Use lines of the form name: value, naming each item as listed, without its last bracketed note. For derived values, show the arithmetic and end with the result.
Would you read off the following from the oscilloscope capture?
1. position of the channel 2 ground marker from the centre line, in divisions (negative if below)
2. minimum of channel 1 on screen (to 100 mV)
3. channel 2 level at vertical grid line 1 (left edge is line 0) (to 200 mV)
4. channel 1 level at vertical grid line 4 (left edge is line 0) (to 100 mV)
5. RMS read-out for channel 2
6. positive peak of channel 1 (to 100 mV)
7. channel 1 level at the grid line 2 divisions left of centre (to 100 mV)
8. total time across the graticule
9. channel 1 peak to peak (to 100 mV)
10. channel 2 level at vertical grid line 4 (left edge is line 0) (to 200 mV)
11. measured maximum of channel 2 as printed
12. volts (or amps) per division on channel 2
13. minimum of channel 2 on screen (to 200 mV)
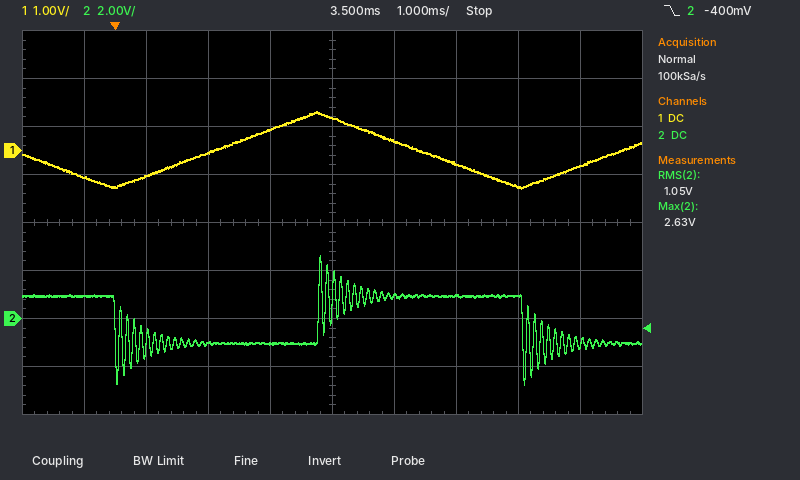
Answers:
position of the channel 2 ground marker from the centre line, in divisions: -2.0 div
minimum of channel 1 on screen: -800 mV
channel 2 level at vertical grid line 1 (left edge is line 0): 1.0 V
channel 1 level at vertical grid line 4 (left edge is line 0): 400 mV
RMS read-out for channel 2: 1.05 V
positive peak of channel 1: 800 mV
channel 1 level at the grid line 2 divisions left of centre: 0.0 V
total time across the graticule: 10 ms
channel 1 peak to peak: 800 mV − (-800 mV) = 1.6 V
channel 2 level at vertical grid line 4 (left edge is line 0): -1.0 V
measured maximum of channel 2 as printed: 2.63 V
volts (or amps) per division on channel 2: 2 V
minimum of channel 2 on screen: -2.8 V
